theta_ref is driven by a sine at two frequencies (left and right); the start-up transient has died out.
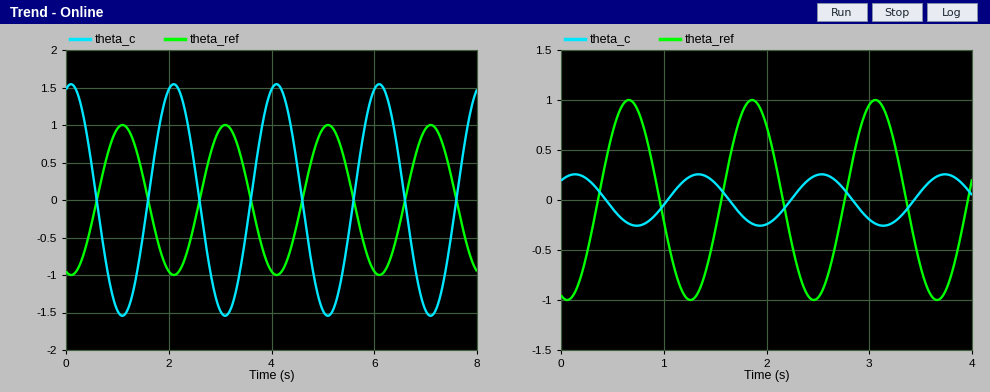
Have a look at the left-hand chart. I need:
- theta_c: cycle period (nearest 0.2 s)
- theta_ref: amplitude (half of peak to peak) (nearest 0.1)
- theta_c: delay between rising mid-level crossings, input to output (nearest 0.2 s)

2.0 s
1.0
1.0 s
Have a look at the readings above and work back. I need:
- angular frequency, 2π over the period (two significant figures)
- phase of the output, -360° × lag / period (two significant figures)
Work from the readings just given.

3.1 rad/s
-180°
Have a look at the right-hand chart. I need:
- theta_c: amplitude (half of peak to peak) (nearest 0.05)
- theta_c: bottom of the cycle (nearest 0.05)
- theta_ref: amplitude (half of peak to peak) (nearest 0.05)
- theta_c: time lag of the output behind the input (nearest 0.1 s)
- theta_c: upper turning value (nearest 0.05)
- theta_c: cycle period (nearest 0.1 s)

0.25
-0.25
1.00
0.7 s
0.25
1.2 s
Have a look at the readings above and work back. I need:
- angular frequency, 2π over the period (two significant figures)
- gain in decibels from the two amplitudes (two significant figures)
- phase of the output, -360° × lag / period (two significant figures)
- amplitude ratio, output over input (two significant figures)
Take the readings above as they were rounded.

5.2 rad/s
-12 dB
-210°
0.25
